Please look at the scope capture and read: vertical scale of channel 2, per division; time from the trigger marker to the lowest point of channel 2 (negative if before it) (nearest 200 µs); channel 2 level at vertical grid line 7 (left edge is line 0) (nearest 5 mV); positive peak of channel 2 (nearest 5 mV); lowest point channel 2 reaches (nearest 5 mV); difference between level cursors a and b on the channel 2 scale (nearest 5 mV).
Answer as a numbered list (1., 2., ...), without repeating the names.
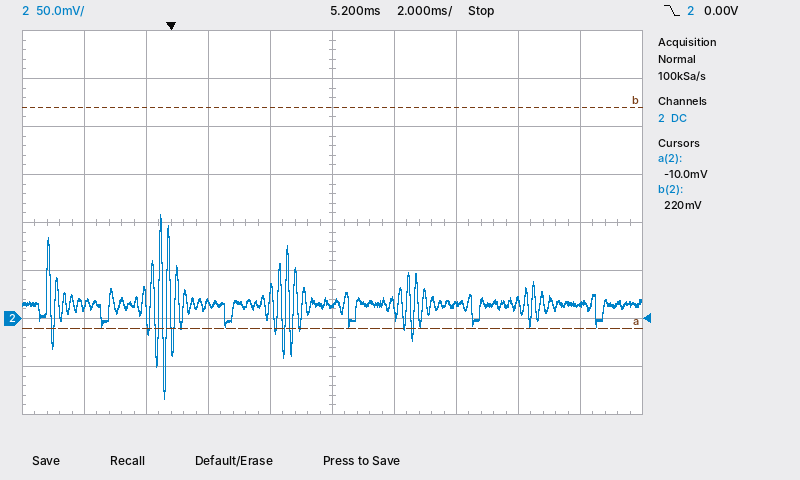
1. 50 mV
2. -200 µs
3. 15 mV
4. 110 mV
5. -85 mV
6. 230 mV
